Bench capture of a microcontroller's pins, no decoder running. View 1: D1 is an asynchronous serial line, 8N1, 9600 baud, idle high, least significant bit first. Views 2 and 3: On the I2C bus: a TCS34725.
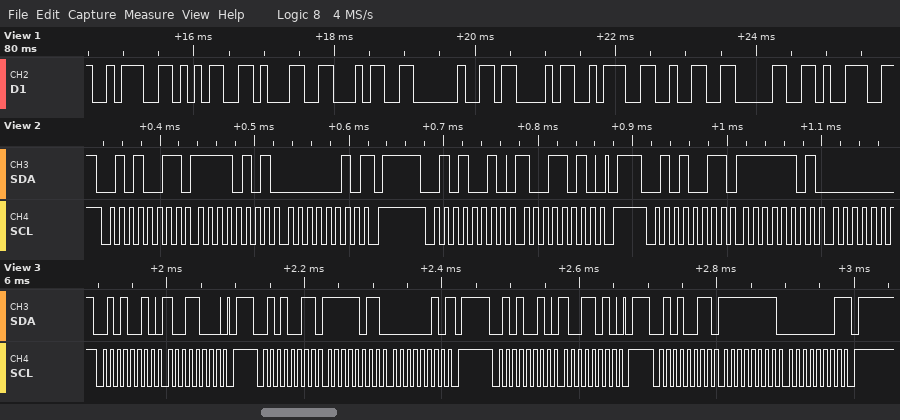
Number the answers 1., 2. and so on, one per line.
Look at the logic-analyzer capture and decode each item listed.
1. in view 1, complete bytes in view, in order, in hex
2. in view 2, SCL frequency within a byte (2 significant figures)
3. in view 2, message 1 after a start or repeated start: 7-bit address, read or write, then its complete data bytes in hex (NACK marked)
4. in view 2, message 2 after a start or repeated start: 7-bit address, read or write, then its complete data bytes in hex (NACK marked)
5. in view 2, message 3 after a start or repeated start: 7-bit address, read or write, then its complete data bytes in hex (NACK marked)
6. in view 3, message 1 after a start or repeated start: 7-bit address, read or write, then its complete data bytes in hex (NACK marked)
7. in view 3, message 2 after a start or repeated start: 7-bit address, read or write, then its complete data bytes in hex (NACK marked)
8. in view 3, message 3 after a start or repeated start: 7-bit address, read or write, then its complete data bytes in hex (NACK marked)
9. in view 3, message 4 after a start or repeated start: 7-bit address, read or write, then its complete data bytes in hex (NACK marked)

1. 0x3A 0x35 0x31 0x34 0x20 0x43 0x3A 0x32 0x30 0x39
2. 100 kHz
3. 0x29 read: F5 02 NACK
4. 0x29 write: 9A
5. 0x29 read: FD
6. 0x29 write: 98
7. 0x29 read: FB 02 NACK
8. 0x29 write: 9A
9. 0x29 read: FF 01 NACK
